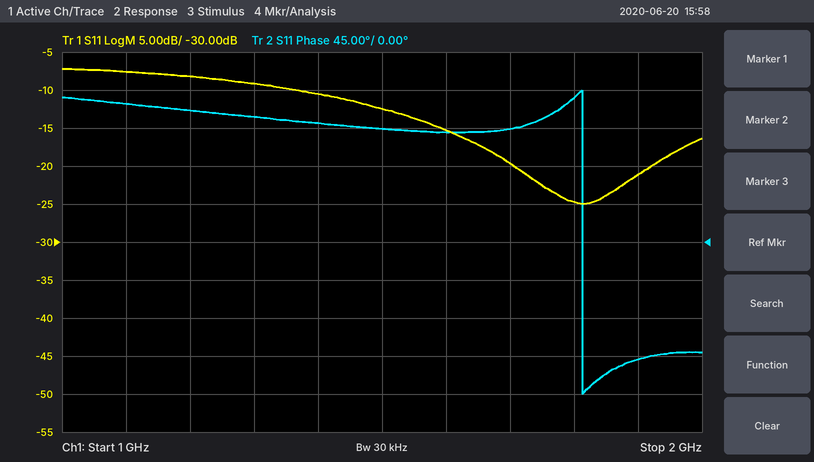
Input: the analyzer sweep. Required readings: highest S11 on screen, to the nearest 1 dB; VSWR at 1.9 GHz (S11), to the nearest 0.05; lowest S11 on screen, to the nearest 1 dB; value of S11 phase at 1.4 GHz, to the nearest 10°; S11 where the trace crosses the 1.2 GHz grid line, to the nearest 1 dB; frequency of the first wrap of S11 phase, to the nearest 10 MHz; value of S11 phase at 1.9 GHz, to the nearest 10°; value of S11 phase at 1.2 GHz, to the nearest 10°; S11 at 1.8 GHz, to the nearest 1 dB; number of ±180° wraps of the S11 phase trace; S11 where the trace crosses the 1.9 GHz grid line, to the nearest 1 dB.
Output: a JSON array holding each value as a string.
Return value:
["-7 dB", "1.20", "-25 dB", "140°", "-8 dB", "1.81 GHz", "-140°", "160°", "-25 dB", "1", "-21 dB"]
